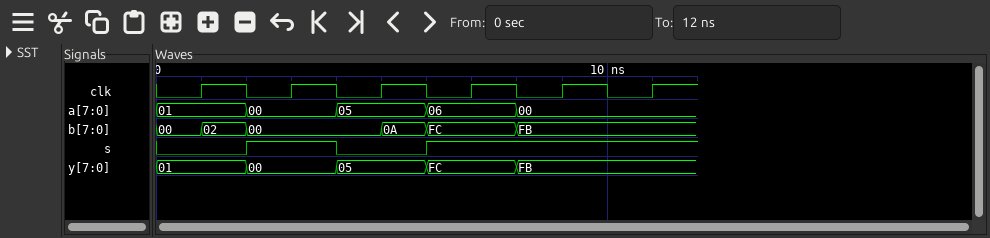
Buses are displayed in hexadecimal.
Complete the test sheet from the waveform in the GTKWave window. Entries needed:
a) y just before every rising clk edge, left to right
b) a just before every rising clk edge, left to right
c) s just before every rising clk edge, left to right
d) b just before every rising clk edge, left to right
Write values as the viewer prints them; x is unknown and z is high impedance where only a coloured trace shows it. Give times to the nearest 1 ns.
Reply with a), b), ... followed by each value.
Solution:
a) 01, 00, 05, FC, FB, FB
b) 01, 00, 05, 06, 00, 00
c) 0 1 0 1 1 1
d) 00, 00, 00, FC, FB, FB
